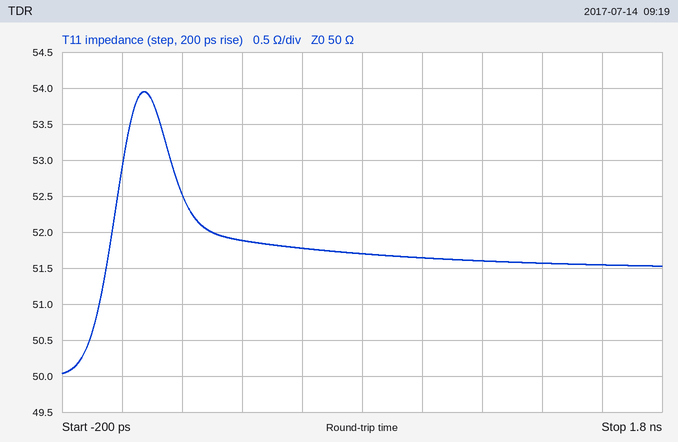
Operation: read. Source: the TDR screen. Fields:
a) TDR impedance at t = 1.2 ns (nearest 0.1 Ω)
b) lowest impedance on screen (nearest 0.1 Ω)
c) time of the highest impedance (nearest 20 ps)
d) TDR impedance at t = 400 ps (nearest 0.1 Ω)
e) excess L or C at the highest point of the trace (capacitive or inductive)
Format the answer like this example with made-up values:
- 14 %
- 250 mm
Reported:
- 51.6 Ω
- 50.0 Ω
- 80 ps
- 51.9 Ω
- inductive
